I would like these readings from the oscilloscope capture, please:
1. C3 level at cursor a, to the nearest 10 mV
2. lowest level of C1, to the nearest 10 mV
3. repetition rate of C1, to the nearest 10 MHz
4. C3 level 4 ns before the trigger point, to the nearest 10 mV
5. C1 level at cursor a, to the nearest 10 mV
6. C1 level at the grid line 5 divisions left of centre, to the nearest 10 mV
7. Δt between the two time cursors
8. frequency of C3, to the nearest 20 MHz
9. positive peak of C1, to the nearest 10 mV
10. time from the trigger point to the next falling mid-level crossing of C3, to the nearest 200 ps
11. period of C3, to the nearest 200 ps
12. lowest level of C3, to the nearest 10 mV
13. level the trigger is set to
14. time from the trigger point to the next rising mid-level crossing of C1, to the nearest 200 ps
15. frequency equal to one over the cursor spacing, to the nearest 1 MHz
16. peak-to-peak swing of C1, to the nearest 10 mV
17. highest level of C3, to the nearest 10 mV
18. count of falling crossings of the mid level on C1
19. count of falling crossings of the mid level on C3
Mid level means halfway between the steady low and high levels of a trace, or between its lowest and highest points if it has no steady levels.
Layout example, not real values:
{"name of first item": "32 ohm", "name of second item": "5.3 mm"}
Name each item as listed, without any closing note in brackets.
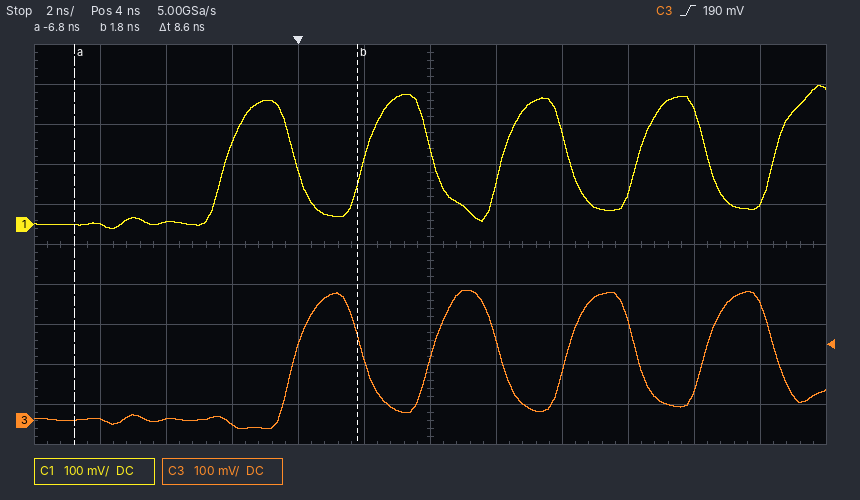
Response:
{"C3 level at cursor a, to the nearest 10 mV": "0 mV", "lowest level of C1, to the nearest 10 mV": "-10 mV", "repetition rate of C1, to the nearest 10 MHz": "240 MHz", "C3 level 4 ns before the trigger point, to the nearest 10 mV": "0 mV", "C1 level at cursor a, to the nearest 10 mV": "0 mV", "C1 level at the grid line 5 divisions left of centre, to the nearest 10 mV": "0 mV", "Δt between the two time cursors": "8.6 ns", "frequency of C3, to the nearest 20 MHz": "240 MHz", "positive peak of C1, to the nearest 10 mV": "350 mV", "time from the trigger point to the next falling mid-level crossing of C3, to the nearest 200 ps": "2.0 ns", "period of C3, to the nearest 200 ps": "4.2 ns", "lowest level of C3, to the nearest 10 mV": "-20 mV", "level the trigger is set to": "190 mV", "time from the trigger point to the next rising mid-level crossing of C1, to the nearest 200 ps": "2.0 ns", "frequency equal to one over the cursor spacing, to the nearest 1 MHz": "116 MHz", "peak-to-peak swing of C1, to the nearest 10 mV": "360 mV", "highest level of C3, to the nearest 10 mV": "330 mV", "count of falling crossings of the mid level on C1": "4", "count of falling crossings of the mid level on C3": "4"}
